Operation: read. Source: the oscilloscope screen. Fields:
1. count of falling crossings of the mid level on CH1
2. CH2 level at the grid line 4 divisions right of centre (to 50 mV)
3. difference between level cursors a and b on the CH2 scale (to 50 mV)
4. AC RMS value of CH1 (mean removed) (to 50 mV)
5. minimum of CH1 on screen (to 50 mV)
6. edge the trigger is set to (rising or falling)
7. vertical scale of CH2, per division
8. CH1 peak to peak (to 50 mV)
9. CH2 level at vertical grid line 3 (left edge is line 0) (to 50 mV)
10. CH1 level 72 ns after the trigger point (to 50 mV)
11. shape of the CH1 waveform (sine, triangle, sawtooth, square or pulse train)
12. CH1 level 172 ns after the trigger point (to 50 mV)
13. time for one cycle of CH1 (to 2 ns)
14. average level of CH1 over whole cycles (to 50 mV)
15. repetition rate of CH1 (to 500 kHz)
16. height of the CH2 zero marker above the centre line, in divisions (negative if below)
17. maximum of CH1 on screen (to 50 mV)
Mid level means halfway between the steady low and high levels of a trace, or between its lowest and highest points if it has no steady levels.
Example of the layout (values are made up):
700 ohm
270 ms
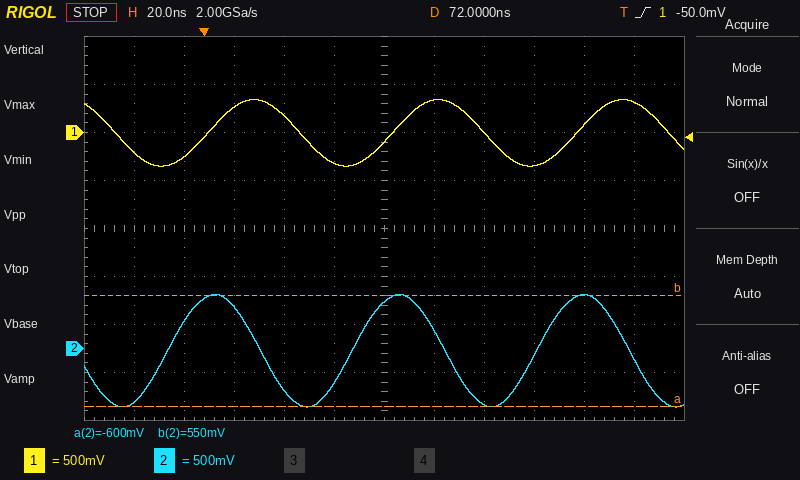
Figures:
4
550 mV
1.15 V
250 mV
-350 mV
rising
500 mV
700 mV
450 mV
-100 mV
sine
300 mV
74 ns
0 mV
13.5 MHz
-2.5 div
350 mV
